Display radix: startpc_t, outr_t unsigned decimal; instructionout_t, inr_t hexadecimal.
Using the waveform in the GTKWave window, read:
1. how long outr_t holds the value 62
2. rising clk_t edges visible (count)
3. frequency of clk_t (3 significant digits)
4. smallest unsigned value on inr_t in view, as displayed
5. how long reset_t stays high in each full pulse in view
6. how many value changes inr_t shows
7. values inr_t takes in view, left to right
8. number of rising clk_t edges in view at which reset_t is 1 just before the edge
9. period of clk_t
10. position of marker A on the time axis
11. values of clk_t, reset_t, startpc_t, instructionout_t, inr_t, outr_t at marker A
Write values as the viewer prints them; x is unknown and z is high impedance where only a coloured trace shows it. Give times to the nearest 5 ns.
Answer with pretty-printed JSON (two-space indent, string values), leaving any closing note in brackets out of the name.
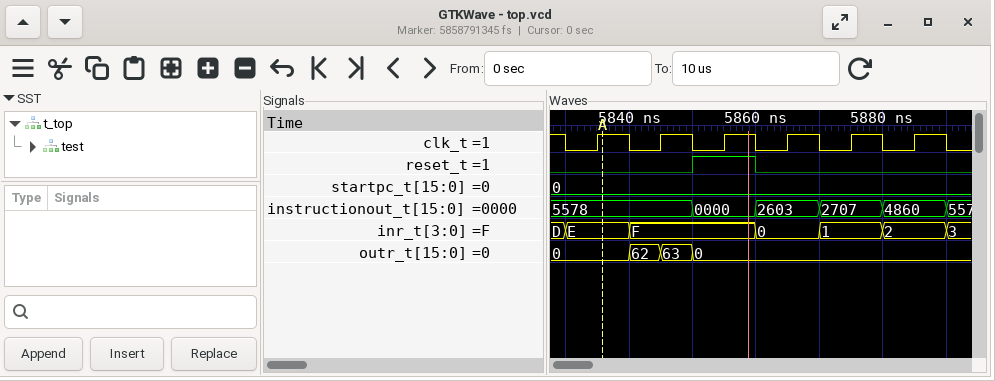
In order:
{
  "how long outr_t holds the value 62": "5 ns",
  "rising clk_t edges visible": "6",
  "frequency of clk_t": "100 MHz",
  "smallest unsigned value on inr_t in view, as displayed": "0",
  "how long reset_t stays high in each full pulse in view": "10 ns",
  "how many value changes inr_t shows": "6",
  "values inr_t takes in view, left to right": "D, E, F, 0, 1, 2, 3",
  "number of rising clk_t edges in view at which reset_t is 1 just before the edge": "1",
  "period of clk_t": "10 ns",
  "position of marker A on the time axis": "5835 ns",
  "values of clk_t, reset_t, startpc_t, instructionout_t, inr_t, outr_t at marker A": "clk_t=1, reset_t=0, startpc_t=0, instructionout_t=5578, inr_t=E, outr_t=0"
}
